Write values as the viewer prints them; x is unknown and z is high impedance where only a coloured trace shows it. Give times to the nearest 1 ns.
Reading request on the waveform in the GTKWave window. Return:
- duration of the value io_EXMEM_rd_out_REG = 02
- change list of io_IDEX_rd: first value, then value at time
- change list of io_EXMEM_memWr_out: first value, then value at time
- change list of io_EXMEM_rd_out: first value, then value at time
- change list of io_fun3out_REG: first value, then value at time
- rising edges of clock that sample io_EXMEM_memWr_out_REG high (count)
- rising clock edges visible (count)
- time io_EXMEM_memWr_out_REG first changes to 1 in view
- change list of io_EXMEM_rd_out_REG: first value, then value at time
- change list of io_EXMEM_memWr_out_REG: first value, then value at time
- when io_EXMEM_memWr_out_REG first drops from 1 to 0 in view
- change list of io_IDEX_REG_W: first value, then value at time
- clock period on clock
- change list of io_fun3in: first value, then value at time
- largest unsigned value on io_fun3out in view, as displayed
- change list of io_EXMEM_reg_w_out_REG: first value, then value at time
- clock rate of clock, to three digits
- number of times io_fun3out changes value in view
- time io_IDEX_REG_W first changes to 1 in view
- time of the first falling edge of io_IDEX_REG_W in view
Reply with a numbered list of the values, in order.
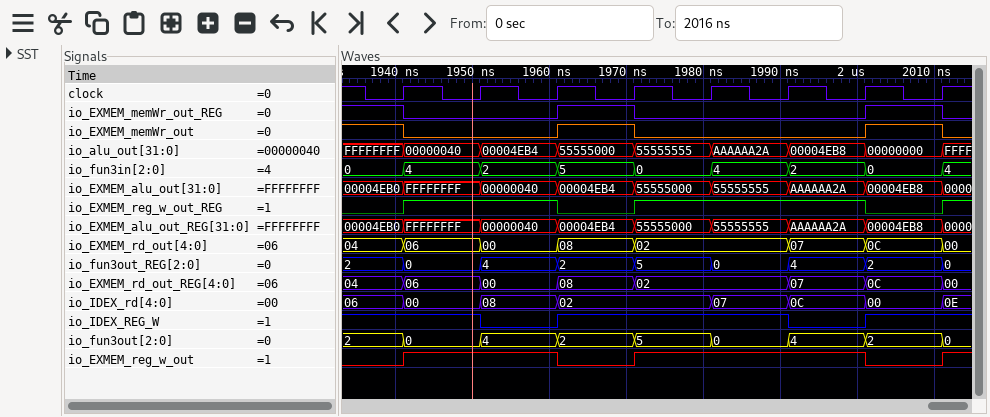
1. 20 ns
2. 06, 00 at 1941 ns, 08 at 1951 ns, 02 at 1961 ns, 07 at 1981 ns, 0C at 1991 ns, 00 at 2001 ns, 0E at 2011 ns
3. 1, 0 at 1941 ns, 1 at 1961 ns, 0 at 1971 ns, 1 at 2001 ns, 0 at 2011 ns
4. 04, 06 at 1941 ns, 00 at 1951 ns, 08 at 1961 ns, 02 at 1971 ns, 07 at 1991 ns, 0C at 2001 ns, 00 at 2011 ns
5. 2, 0 at 1941 ns, 4 at 1951 ns, 2 at 1961 ns, 5 at 1971 ns, 0 at 1981 ns, 4 at 1991 ns, 2 at 2001 ns, 0 at 2011 ns
6. 3
7. 8
8. 1961 ns
9. 04, 06 at 1941 ns, 00 at 1951 ns, 08 at 1961 ns, 02 at 1971 ns, 07 at 1991 ns, 0C at 2001 ns, 00 at 2011 ns
10. 1, 0 at 1941 ns, 1 at 1961 ns, 0 at 1971 ns, 1 at 2001 ns, 0 at 2011 ns
11. 1941 ns
12. 1, 0 at 1951 ns, 1 at 1961 ns, 0 at 1991 ns, 1 at 2001 ns
13. 10 ns
14. 0, 4 at 1941 ns, 2 at 1951 ns, 5 at 1961 ns, 0 at 1971 ns, 4 at 1981 ns, 2 at 1991 ns, 0 at 2001 ns, 4 at 2011 ns
15. 5
16. 0, 1 at 1941 ns, 0 at 1961 ns, 1 at 1971 ns, 0 at 2001 ns, 1 at 2011 ns
17. 100 MHz
18. 8
19. 1961 ns
20. 1951 ns
